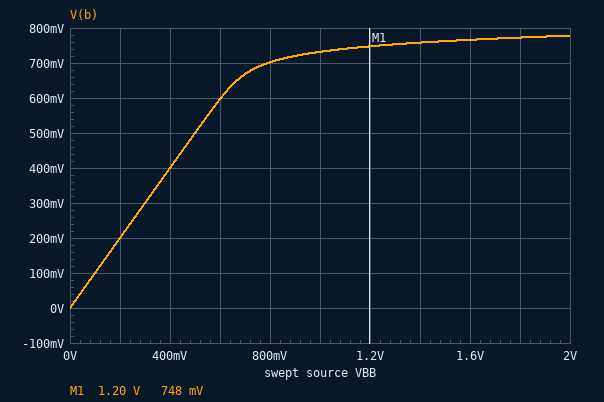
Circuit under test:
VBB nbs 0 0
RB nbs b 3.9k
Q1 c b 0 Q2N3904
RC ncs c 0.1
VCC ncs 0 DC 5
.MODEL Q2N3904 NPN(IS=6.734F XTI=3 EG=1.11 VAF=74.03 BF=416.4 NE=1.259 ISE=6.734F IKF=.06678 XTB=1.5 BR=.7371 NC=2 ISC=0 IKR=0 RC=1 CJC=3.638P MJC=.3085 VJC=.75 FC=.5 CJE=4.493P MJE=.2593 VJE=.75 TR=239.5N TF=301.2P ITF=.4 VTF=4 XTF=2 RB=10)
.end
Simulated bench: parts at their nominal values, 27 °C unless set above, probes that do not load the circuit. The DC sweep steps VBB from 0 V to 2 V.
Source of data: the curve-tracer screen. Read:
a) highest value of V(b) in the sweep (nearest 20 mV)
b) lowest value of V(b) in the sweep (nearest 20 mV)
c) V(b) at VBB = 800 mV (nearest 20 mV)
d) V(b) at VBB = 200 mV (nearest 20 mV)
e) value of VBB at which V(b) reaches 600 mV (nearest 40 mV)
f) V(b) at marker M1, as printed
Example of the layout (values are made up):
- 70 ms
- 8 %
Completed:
- 780 mV
- 0 V
- 700 mV
- 200 mV
- 600 mV
- 748 mV
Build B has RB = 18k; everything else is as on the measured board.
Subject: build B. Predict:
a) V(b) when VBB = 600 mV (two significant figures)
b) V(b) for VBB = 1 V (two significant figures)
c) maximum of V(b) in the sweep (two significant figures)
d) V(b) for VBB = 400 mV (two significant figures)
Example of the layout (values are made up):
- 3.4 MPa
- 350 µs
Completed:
- 590 mV
- 690 mV
- 730 mV
- 400 mV
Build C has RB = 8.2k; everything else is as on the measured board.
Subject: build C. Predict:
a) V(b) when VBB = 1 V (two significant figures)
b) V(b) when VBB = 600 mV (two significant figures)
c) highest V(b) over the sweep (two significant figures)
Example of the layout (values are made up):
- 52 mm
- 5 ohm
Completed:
- 710 mV
- 590 mV
- 760 mV
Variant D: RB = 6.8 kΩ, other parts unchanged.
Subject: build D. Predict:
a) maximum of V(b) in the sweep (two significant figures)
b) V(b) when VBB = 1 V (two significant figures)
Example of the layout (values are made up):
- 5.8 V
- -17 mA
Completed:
- 760 mV
- 720 mV
